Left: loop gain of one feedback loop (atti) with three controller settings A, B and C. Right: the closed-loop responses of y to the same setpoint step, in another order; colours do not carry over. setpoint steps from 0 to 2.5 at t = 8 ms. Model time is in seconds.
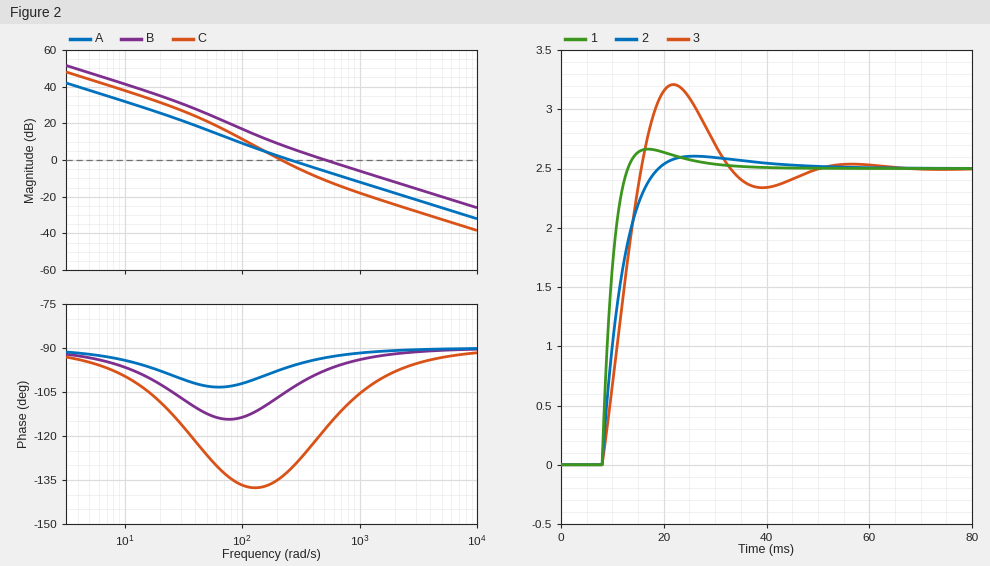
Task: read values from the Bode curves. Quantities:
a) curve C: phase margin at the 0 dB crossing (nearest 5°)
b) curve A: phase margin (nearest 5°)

45°
85°
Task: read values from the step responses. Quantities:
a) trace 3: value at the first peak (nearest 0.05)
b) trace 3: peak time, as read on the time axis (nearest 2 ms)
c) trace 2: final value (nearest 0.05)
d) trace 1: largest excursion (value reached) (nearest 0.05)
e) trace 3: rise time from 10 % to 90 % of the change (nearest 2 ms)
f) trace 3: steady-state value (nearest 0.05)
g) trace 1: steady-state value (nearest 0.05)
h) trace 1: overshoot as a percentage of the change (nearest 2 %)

3.20
22 ms
2.50
2.65
6 ms
2.50
2.50
6 %
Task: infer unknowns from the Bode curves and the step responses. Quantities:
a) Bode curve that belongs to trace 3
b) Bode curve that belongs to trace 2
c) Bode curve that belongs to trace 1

C
A
B
